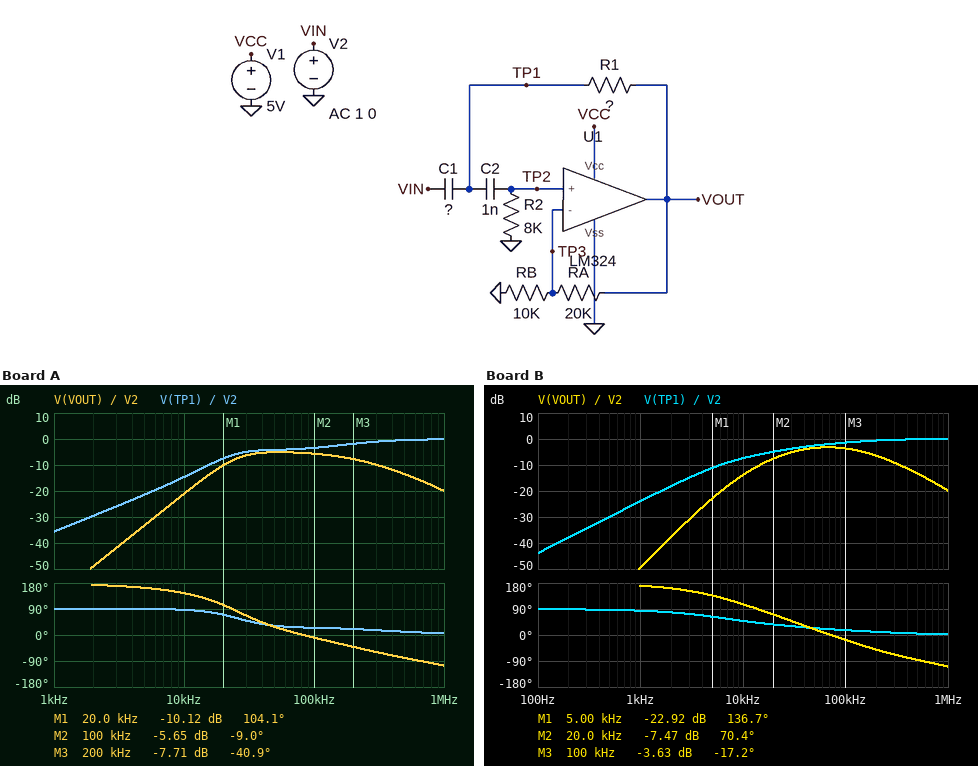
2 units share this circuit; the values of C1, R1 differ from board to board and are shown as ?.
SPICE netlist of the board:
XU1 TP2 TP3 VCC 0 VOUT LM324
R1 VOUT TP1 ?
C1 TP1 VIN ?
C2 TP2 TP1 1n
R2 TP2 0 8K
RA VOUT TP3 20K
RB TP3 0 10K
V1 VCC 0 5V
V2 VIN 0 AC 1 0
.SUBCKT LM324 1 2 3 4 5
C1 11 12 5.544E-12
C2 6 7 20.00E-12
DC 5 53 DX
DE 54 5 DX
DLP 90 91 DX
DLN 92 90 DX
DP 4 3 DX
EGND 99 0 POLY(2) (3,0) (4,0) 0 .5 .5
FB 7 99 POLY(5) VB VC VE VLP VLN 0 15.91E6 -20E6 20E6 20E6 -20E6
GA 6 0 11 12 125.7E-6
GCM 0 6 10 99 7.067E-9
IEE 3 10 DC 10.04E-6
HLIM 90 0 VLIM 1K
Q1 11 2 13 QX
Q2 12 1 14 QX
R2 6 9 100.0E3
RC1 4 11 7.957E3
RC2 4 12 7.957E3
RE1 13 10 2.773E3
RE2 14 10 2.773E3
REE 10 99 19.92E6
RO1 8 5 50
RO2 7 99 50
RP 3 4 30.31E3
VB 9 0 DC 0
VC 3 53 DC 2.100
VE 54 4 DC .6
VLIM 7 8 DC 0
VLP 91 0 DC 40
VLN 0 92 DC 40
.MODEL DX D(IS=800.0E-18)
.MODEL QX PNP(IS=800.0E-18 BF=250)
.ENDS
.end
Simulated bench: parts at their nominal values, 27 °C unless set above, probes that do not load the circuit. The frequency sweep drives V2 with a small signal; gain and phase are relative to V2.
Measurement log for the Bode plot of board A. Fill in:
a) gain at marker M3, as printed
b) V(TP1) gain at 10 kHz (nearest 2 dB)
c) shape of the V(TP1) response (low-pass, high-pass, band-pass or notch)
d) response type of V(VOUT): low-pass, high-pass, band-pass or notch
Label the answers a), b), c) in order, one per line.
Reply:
a) -7.71 dB
b) -14 dB
c) high-pass
d) band-pass
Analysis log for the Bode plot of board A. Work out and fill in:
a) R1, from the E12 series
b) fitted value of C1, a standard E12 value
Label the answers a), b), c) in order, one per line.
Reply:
a) 5.6 kΩ
b) 470 pF
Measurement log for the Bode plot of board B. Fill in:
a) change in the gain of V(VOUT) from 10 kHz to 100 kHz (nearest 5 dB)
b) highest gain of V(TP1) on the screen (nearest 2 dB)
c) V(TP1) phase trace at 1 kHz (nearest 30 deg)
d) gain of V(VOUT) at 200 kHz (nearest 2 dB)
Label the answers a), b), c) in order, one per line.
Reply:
a) 10 dB
b) 0 dB
c) 90 deg
d) -6 dB
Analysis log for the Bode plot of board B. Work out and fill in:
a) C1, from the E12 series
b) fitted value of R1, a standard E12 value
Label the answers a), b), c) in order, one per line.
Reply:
a) 680 pF
b) 15 kΩ
